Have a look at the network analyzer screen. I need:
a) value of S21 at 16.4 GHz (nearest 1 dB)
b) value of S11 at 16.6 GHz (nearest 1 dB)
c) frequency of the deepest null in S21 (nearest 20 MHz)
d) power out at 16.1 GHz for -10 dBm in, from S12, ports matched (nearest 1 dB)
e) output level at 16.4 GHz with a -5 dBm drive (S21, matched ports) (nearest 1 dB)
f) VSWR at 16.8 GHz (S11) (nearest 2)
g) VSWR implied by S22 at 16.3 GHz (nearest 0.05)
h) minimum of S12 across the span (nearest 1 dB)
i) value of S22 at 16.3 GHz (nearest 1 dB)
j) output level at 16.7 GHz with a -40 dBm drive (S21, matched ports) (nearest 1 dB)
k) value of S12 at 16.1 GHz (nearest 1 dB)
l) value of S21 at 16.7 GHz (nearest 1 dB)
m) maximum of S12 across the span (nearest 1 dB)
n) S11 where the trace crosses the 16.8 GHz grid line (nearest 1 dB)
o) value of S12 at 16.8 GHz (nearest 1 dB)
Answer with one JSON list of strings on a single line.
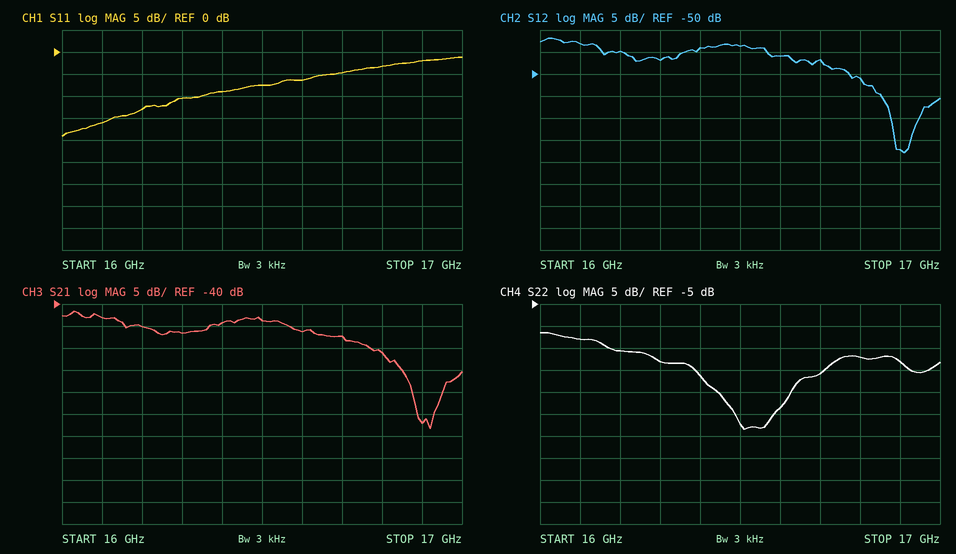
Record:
["-44 dB", "-6 dB", "16.92 GHz", "-53 dBm", "-49 dBm", "6", "1.30", "-68 dB", "-18 dB", "-87 dBm", "-43 dB", "-47 dB", "-42 dB", "-3 dB", "-51 dB"]
